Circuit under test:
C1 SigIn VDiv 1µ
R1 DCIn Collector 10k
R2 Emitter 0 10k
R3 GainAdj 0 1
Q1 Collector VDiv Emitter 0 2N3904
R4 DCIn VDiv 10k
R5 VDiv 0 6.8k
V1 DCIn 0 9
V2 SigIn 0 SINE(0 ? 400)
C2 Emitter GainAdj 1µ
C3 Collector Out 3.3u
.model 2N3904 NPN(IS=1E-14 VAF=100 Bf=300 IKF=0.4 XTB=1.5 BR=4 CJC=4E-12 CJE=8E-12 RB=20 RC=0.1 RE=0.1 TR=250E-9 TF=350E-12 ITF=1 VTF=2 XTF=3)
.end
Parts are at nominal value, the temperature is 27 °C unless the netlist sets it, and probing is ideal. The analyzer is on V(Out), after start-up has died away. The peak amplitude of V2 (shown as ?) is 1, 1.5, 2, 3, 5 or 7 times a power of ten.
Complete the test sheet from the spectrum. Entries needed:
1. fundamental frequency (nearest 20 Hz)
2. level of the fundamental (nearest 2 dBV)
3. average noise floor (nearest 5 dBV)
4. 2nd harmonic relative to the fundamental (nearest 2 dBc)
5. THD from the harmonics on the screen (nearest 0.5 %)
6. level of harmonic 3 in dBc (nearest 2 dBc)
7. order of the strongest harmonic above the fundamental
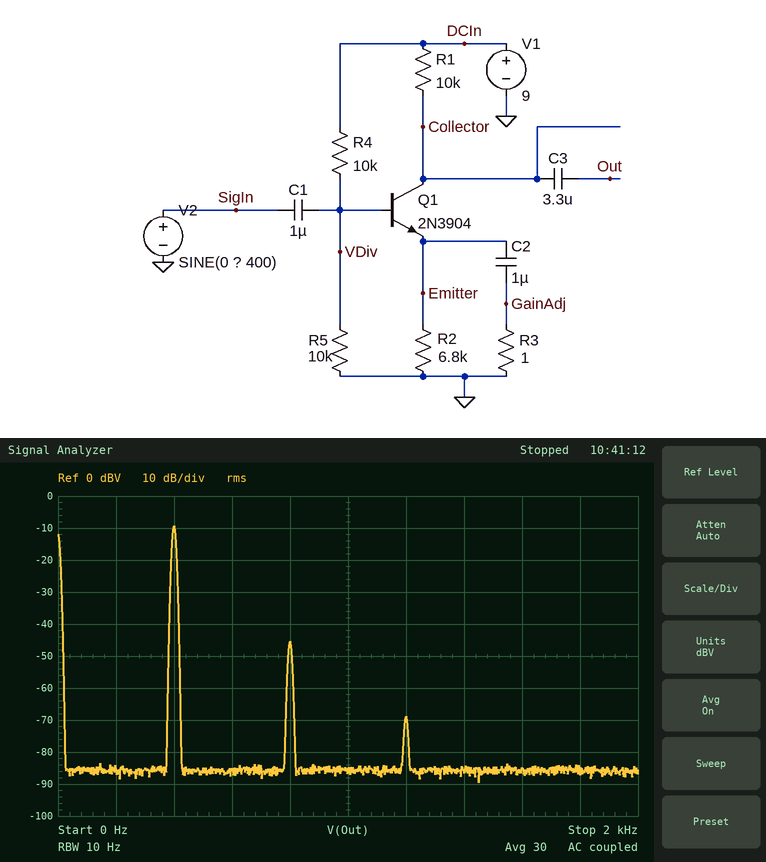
400 Hz
-10 dBV
-85 dBV
-36 dBc
1.5 %
-60 dBc
2
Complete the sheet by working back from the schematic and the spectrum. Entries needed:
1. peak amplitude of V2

20 mV
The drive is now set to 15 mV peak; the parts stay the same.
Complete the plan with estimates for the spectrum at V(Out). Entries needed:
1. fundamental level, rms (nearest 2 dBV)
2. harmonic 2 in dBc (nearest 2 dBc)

-12 dBV
-38 dBc
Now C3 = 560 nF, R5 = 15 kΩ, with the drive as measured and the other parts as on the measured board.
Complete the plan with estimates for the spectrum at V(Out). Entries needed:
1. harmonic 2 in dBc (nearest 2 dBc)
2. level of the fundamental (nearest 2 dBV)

-10 dBc
-34 dBV
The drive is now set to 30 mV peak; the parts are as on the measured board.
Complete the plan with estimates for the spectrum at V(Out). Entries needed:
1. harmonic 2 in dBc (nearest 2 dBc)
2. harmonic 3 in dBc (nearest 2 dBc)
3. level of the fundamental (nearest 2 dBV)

-32 dBc
-52 dBc
-6 dBV
